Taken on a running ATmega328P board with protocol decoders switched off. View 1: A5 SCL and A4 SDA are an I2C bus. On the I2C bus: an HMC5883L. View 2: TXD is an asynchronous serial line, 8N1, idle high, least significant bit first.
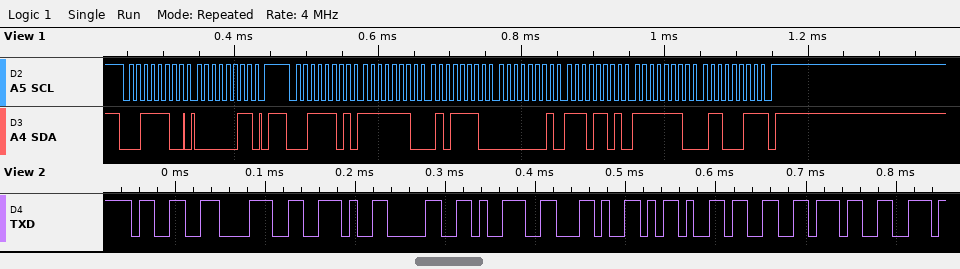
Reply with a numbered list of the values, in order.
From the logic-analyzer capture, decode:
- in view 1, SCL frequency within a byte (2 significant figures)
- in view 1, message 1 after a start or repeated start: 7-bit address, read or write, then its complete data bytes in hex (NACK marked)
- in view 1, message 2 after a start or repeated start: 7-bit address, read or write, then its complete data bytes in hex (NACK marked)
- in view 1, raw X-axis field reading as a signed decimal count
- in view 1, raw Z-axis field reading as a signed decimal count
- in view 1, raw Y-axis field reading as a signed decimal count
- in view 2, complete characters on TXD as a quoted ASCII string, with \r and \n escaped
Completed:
1. 100 kHz
2. 0x1E write: 03
3. 0x1E read: FE 5E 01 ED FE 63 NACK
4. -418
5. 493
6. -413
7. "38.09,-37"
